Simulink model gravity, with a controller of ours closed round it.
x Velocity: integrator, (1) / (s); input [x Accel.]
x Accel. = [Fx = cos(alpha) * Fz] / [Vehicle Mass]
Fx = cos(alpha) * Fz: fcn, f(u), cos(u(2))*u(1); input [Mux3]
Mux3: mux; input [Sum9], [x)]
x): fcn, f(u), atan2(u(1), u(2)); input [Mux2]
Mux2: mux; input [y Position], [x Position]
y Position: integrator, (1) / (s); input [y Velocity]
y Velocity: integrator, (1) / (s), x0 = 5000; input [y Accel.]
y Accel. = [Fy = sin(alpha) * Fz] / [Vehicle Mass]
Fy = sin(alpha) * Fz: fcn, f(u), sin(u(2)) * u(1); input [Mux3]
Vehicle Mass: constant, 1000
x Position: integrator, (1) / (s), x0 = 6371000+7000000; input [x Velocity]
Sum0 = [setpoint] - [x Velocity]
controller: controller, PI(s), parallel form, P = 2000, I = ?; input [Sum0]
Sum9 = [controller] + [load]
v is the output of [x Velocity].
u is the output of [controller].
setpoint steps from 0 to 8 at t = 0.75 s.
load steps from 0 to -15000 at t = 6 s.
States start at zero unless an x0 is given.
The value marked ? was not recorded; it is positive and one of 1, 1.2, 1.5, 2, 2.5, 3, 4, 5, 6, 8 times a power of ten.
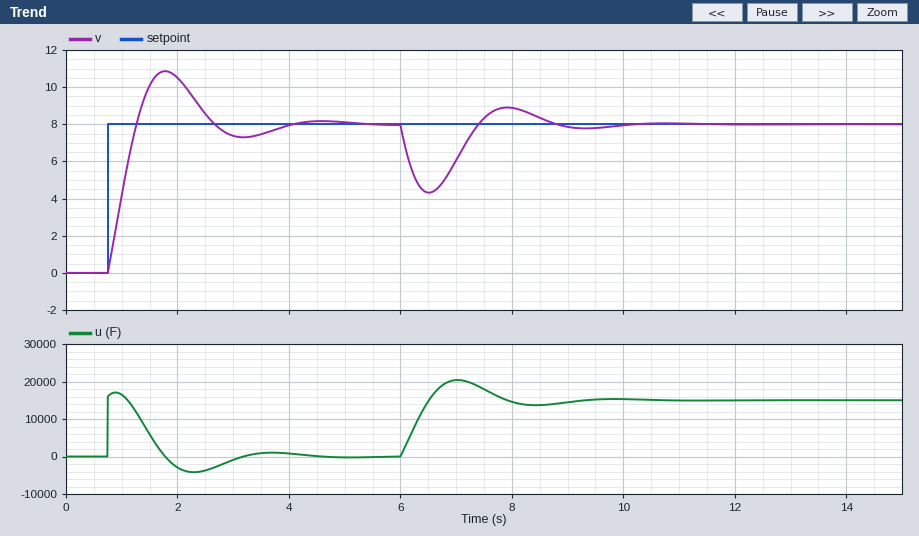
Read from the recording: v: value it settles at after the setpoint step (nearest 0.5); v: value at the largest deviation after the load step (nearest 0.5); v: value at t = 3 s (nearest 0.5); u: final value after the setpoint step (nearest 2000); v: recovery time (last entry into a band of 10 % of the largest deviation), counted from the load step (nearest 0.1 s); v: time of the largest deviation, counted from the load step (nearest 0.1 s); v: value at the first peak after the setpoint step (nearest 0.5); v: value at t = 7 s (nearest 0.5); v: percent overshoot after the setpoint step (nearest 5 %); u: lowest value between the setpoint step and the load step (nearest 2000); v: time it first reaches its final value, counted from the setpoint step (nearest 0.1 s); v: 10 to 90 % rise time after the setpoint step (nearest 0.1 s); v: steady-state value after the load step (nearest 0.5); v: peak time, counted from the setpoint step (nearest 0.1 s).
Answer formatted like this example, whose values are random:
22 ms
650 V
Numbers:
8.0
4.5
7.5
0
2.5 s
0.5 s
11.0
6.0
35 %
-4000
0.5 s
0.4 s
8.0
1.0 s
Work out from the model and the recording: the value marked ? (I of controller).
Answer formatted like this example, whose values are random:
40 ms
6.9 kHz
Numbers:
6000
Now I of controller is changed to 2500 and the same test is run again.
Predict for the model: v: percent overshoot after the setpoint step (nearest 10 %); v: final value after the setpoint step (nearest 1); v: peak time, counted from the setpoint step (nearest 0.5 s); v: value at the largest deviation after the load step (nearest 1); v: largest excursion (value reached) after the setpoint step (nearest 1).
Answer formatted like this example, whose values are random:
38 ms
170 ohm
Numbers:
20 %
8
1.5 s
3
10
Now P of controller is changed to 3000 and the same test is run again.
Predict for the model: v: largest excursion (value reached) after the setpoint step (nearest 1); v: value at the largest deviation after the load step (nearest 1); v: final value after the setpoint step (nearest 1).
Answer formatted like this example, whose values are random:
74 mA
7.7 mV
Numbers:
10
5
8
